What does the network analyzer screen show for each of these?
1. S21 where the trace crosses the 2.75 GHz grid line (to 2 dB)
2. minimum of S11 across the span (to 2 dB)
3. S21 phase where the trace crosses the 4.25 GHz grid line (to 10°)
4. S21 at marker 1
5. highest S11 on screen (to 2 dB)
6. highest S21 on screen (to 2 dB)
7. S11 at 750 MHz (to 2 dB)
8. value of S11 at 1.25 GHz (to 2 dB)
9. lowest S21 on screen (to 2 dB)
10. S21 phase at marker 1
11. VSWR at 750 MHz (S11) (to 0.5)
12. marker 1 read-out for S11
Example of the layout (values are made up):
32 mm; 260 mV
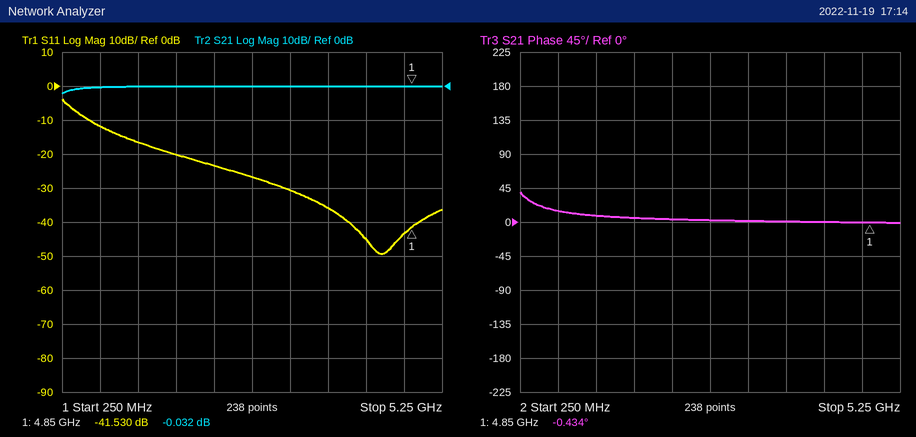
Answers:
0 dB; -50 dB; 0°; -0.032 dB; -4 dB; 0 dB; -12 dB; -16 dB; -2 dB; -0.434°; 1.5; -41.530 dB
